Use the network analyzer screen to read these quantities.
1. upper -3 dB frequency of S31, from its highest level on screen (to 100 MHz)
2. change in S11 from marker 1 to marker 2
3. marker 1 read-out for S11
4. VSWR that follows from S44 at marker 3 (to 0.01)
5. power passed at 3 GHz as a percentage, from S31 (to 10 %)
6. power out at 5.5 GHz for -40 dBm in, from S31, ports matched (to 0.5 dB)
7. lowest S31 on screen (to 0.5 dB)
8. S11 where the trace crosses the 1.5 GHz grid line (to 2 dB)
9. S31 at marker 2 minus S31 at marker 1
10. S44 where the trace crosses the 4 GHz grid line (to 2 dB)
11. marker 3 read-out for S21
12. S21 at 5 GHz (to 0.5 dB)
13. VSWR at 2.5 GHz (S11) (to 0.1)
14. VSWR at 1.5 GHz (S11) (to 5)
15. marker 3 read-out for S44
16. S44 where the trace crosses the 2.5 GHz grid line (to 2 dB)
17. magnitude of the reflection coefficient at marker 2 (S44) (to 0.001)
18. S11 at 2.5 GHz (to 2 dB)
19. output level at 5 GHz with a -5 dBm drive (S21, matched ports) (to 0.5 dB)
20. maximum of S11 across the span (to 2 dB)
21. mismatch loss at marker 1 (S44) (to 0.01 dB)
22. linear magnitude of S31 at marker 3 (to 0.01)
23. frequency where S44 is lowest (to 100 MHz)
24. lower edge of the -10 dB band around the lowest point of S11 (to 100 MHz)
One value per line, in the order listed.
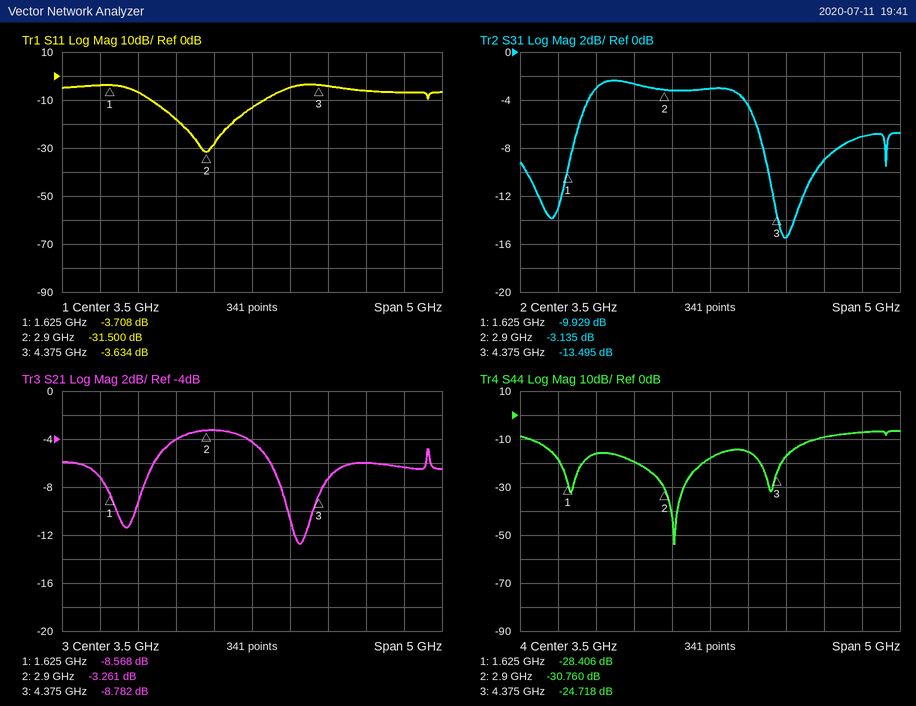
4.1 GHz
-27.792 dB
-3.708 dB
1.12
50 %
-47.0 dBm
-15.5 dB
-4 dB
6.794 dB
-16 dB
-8.782 dB
-6.0 dB
1.3
5
-24.718 dB
-20 dB
0.029
-18 dB
-11.0 dBm
-4 dB
0.01 dB
0.21
3.0 GHz
2.2 GHz
